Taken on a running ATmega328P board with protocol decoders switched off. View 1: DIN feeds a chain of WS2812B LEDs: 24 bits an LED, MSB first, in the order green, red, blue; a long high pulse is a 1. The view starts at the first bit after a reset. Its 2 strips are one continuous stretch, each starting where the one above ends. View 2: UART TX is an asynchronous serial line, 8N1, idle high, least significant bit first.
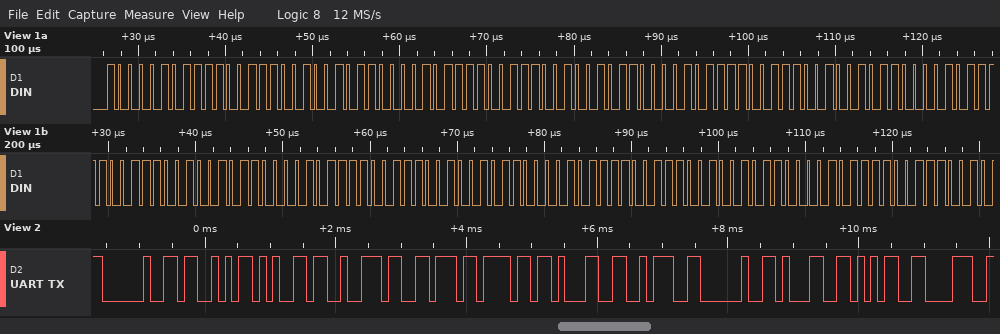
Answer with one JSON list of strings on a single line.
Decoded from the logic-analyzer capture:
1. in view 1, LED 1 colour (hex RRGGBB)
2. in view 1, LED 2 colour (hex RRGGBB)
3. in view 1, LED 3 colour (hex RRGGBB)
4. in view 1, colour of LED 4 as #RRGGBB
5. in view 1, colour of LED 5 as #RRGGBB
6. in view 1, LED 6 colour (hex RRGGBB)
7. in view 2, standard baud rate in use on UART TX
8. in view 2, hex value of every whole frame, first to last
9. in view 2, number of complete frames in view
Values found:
["#E78525", "#E78525", "#E78525", "#E78525", "#E78525", "#E78525", "9600 baud", "20 53 65 72 76 6F 31 3A 20 31 35 38", "12"]
